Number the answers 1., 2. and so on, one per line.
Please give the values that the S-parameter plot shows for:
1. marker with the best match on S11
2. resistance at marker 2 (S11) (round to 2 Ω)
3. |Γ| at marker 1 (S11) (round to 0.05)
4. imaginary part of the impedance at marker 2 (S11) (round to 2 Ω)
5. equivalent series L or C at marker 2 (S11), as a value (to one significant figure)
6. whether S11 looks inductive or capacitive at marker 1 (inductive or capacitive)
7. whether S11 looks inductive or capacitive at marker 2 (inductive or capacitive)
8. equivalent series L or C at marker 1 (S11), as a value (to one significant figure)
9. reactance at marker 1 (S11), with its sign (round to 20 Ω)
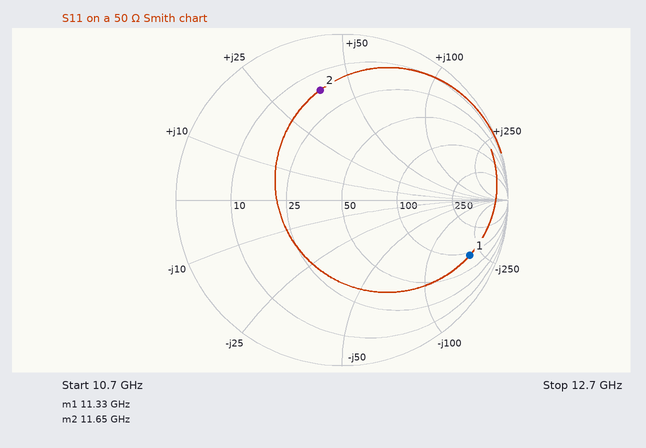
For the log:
1. marker 2
2. 16 Ω
3. 0.85
4. +38 Ω
5. 500 pH
6. capacitive
7. inductive
8. 70 fF
9. -200 Ω
